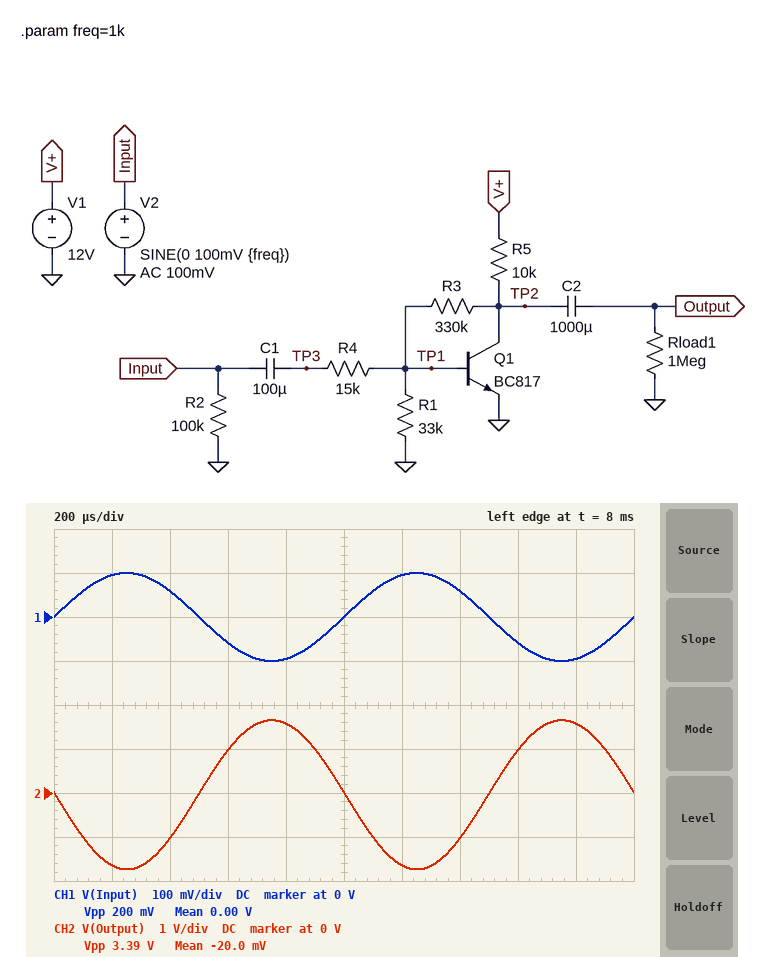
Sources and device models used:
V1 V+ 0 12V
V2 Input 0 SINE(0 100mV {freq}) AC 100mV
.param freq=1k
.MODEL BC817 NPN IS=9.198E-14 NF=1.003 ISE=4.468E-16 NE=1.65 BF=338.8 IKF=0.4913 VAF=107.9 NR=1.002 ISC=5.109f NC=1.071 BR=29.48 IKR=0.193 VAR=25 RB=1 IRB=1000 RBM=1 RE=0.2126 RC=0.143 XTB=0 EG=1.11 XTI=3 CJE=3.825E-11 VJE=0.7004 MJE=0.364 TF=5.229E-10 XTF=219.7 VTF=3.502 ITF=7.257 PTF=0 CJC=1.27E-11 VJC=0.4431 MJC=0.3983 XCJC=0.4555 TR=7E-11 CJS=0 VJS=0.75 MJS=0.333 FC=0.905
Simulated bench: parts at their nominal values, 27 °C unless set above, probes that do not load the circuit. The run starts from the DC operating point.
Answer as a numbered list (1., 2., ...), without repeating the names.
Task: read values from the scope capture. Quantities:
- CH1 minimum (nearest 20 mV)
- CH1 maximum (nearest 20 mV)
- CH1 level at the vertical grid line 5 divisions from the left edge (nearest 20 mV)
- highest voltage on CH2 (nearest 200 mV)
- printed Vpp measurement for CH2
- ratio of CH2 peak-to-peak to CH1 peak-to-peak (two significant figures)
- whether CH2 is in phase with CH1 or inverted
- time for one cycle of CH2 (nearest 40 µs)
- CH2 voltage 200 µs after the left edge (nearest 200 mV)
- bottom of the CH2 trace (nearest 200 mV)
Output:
1. -100 mV
2. 100 mV
3. 0 V
4. 1.6 V
5. 3.39 V
6. 17
7. inverted
8. 1.00 ms
9. -1.6 V
10. -1.8 V
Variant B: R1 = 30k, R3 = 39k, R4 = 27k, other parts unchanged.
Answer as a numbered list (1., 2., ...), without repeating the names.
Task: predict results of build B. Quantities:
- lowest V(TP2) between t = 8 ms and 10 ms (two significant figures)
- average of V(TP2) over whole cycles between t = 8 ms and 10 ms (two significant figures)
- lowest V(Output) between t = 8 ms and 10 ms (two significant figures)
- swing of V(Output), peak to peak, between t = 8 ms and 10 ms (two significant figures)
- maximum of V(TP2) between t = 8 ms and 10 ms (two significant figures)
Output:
1. 1.4 V
2. 1.5 V
3. -140 mV
4. 280 mV
5. 1.6 V
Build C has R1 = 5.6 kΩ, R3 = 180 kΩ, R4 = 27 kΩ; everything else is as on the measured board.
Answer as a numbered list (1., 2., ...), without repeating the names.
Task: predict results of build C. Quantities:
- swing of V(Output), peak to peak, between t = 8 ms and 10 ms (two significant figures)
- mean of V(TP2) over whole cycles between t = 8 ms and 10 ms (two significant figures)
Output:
1. 1.0 mV
2. 11 V
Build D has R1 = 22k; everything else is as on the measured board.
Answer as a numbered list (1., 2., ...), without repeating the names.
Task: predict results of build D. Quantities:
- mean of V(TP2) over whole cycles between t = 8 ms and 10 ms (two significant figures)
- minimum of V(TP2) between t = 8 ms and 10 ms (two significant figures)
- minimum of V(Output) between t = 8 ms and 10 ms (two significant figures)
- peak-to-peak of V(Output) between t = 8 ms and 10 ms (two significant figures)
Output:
1. 9.2 V
2. 7.7 V
3. -1.5 V
4. 2.8 V
